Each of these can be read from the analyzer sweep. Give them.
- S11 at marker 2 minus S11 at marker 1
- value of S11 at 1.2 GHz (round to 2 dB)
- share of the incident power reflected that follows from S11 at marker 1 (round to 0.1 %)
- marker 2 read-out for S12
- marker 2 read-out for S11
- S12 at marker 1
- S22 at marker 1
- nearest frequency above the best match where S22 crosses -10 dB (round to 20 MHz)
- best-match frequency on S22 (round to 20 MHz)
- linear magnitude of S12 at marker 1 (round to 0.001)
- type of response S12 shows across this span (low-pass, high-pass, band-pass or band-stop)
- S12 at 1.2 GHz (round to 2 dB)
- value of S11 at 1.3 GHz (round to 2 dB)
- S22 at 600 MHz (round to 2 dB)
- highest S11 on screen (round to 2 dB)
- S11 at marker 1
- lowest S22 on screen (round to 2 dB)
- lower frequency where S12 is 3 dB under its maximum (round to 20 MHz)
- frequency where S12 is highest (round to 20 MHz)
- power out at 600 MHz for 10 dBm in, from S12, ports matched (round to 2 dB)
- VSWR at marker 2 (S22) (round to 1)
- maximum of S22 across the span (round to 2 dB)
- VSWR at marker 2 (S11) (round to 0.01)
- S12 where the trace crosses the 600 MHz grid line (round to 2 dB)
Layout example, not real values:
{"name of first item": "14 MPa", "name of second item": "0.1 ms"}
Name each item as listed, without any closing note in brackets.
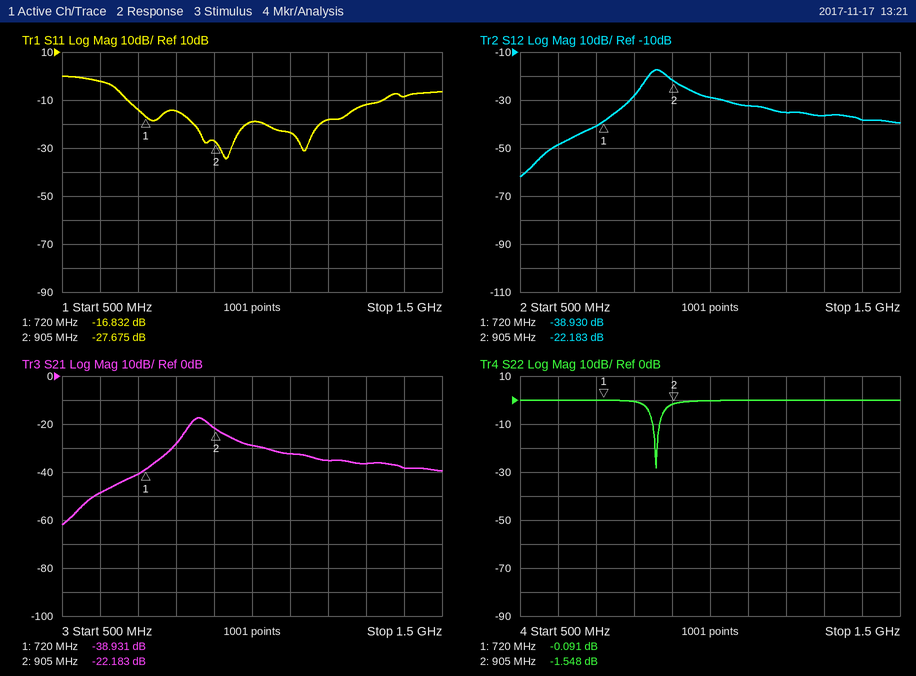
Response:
{"S11 at marker 2 minus S11 at marker 1": "-10.843 dB", "value of S11 at 1.2 GHz": "-18 dB", "share of the incident power reflected that follows from S11 at marker 1": "2.1 %", "marker 2 read-out for S12": "-22.183 dB", "marker 2 read-out for S11": "-27.675 dB", "S12 at marker 1": "-38.930 dB", "S22 at marker 1": "-0.091 dB", "nearest frequency above the best match where S22 crosses -10 dB": "860 MHz", "best-match frequency on S22": "860 MHz", "linear magnitude of S12 at marker 1": "0.011", "type of response S12 shows across this span": "band-pass", "S12 at 1.2 GHz": "-36 dB", "value of S11 at 1.3 GHz": "-12 dB", "S22 at 600 MHz": "0 dB", "highest S11 on screen": "0 dB", "S11 at marker 1": "-16.832 dB", "lowest S22 on screen": "-28 dB", "lower frequency where S12 is 3 dB under its maximum": "840 MHz", "frequency where S12 is highest": "860 MHz", "power out at 600 MHz for 10 dBm in, from S12, ports matched": "-38 dBm", "VSWR at marker 2 (S22)": "11", "maximum of S22 across the span": "0 dB", "VSWR at marker 2 (S11)": "1.09", "S12 where the trace crosses the 600 MHz grid line": "-48 dB"}
